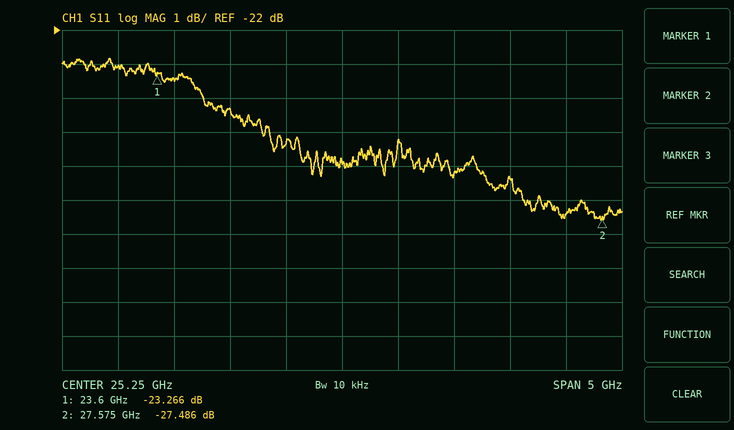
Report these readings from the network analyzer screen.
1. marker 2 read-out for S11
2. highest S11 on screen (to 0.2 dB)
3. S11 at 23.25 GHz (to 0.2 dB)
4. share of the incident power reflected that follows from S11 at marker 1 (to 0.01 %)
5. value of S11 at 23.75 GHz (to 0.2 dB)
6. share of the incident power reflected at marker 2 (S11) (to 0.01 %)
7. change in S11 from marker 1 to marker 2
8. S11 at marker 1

-27.486 dB
-22.8 dB
-23.0 dB
0.47 %
-23.4 dB
0.18 %
-4.220 dB
-23.266 dB
